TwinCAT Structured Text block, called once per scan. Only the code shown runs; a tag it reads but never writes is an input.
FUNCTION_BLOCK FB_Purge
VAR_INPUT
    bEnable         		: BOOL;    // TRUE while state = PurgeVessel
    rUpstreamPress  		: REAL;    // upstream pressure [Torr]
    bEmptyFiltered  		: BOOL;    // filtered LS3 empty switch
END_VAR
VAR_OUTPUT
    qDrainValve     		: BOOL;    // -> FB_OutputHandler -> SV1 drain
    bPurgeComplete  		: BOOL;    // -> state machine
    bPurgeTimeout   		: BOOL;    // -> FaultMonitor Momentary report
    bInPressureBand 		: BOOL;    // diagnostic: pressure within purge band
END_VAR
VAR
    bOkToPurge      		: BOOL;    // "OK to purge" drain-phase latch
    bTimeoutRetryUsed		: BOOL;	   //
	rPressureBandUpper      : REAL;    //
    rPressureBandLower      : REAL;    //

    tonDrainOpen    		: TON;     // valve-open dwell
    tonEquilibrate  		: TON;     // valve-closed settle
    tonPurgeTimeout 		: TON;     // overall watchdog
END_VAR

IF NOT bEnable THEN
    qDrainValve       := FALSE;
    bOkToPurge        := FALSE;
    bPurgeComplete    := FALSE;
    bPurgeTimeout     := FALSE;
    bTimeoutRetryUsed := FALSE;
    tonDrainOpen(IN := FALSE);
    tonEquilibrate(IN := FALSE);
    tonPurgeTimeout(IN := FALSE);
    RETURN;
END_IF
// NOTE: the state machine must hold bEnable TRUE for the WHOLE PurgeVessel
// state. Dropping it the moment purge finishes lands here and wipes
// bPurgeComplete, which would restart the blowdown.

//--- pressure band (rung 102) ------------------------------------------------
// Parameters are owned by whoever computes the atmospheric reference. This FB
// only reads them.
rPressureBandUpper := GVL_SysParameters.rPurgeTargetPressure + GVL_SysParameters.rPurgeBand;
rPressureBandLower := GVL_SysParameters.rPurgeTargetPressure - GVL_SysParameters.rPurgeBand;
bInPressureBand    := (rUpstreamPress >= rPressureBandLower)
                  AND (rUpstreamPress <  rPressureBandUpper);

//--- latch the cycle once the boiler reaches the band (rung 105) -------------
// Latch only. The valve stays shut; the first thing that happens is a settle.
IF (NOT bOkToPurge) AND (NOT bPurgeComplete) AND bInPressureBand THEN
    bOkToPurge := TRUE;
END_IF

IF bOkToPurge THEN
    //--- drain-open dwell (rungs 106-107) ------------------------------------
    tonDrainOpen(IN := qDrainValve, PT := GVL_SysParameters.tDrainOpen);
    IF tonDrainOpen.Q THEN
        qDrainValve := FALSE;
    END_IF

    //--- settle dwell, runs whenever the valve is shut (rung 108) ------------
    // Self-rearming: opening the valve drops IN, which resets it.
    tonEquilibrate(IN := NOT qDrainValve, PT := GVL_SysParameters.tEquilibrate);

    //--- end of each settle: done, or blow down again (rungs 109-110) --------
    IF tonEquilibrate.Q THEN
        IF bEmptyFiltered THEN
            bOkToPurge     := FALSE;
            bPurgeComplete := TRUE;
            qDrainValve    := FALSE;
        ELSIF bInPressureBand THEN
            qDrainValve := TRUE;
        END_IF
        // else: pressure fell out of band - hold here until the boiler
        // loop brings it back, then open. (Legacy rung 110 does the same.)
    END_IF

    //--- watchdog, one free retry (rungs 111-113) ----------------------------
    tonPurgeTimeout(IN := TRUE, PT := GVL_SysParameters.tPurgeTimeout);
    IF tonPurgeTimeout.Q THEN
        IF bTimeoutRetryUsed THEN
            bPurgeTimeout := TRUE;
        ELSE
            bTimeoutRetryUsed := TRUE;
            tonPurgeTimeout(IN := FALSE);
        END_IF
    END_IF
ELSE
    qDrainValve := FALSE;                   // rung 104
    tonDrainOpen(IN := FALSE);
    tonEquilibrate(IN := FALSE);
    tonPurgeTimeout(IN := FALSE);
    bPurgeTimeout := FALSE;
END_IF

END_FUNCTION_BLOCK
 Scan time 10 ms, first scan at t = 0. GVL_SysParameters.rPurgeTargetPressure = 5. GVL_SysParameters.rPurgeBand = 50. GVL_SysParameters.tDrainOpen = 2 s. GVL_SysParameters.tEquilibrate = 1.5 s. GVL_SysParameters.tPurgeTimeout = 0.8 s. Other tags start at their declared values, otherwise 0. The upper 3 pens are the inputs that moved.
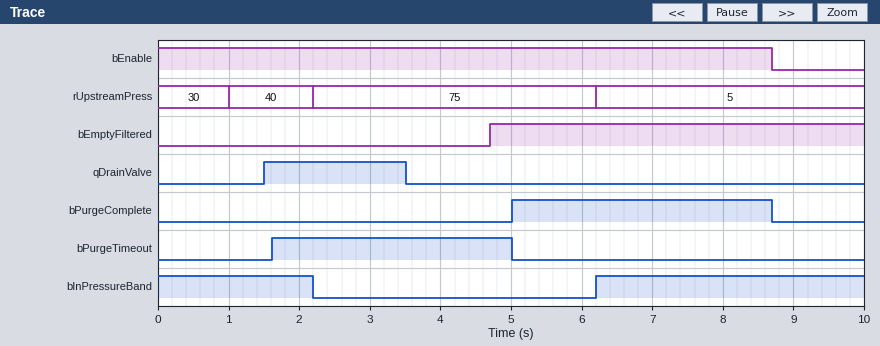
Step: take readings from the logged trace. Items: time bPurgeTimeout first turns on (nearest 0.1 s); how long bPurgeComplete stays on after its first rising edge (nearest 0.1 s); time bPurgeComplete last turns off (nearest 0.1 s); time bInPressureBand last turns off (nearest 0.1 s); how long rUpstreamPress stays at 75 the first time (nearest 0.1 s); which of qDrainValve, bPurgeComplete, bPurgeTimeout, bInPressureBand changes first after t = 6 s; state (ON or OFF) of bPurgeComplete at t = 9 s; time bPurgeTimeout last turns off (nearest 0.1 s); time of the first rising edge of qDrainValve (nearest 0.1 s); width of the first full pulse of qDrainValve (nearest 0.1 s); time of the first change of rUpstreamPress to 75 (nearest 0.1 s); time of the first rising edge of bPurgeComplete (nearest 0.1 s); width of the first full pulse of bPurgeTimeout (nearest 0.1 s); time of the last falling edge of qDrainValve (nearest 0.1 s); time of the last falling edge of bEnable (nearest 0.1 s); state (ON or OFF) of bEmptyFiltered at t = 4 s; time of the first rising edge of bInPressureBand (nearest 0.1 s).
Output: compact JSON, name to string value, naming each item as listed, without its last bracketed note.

{"time bPurgeTimeout first turns on": "1.6 s", "how long bPurgeComplete stays on after its first rising edge": "3.7 s", "time bPurgeComplete last turns off": "8.7 s", "time bInPressureBand last turns off": "2.2 s", "how long rUpstreamPress stays at 75 the first time": "4.0 s", "which of qDrainValve, bPurgeComplete, bPurgeTimeout, bInPressureBand changes first after t = 6 s": "bInPressureBand", "state (ON or OFF) of bPurgeComplete at t = 9 s": "OFF", "time bPurgeTimeout last turns off": "5.0 s", "time of the first rising edge of qDrainValve": "1.5 s", "width of the first full pulse of qDrainValve": "2.0 s", "time of the first change of rUpstreamPress to 75": "2.2 s", "time of the first rising edge of bPurgeComplete": "5.0 s", "width of the first full pulse of bPurgeTimeout": "3.4 s", "time of the last falling edge of qDrainValve": "3.5 s", "time of the last falling edge of bEnable": "8.7 s", "state (ON or OFF) of bEmptyFiltered at t = 4 s": "OFF", "time of the first rising edge of bInPressureBand": "6.2 s"}
